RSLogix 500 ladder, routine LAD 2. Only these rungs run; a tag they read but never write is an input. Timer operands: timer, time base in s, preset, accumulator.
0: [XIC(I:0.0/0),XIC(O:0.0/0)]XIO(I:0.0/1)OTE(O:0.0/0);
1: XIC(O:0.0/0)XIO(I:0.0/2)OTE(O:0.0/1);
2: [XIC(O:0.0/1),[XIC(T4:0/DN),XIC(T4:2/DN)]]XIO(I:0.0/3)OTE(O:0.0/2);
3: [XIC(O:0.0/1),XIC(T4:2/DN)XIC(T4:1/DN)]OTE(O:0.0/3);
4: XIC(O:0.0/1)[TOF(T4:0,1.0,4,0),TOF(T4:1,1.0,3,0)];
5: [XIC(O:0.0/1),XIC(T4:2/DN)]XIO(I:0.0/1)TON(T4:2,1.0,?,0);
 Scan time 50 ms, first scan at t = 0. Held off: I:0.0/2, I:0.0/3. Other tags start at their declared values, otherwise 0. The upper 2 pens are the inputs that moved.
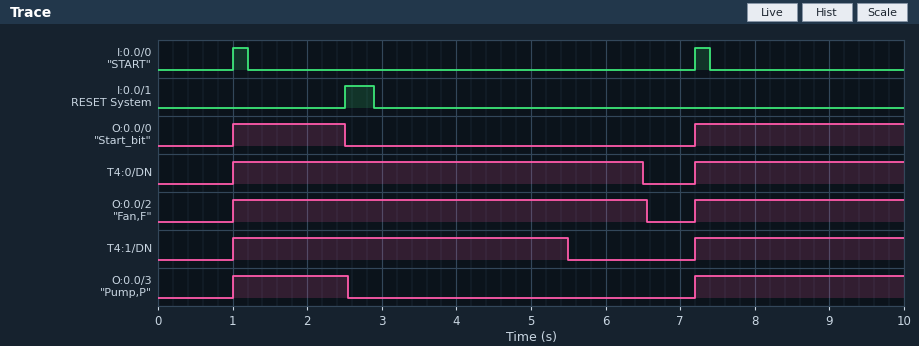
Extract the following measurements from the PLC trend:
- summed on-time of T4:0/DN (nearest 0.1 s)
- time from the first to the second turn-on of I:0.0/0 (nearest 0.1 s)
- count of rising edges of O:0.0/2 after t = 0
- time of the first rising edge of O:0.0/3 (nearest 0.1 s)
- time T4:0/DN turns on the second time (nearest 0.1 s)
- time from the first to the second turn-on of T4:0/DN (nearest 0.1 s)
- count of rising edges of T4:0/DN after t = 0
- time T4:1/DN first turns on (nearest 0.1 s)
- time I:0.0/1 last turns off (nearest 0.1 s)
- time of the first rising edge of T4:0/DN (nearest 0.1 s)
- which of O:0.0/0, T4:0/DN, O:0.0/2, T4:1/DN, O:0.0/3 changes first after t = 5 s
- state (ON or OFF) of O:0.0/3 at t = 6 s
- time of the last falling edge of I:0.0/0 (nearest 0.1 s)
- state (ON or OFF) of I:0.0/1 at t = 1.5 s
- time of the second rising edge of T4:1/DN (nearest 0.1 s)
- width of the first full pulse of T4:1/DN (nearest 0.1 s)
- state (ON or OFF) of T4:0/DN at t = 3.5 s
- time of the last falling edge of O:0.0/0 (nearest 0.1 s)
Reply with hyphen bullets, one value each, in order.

- 8.3 s
- 6.2 s
- 2
- 1.0 s
- 7.2 s
- 6.2 s
- 2
- 1.0 s
- 2.9 s
- 1.0 s
- T4:1/DN
- OFF
- 7.4 s
- OFF
- 7.2 s
- 4.5 s
- ON
- 2.5 s
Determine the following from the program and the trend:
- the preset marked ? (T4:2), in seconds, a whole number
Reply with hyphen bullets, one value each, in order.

- 1 s
